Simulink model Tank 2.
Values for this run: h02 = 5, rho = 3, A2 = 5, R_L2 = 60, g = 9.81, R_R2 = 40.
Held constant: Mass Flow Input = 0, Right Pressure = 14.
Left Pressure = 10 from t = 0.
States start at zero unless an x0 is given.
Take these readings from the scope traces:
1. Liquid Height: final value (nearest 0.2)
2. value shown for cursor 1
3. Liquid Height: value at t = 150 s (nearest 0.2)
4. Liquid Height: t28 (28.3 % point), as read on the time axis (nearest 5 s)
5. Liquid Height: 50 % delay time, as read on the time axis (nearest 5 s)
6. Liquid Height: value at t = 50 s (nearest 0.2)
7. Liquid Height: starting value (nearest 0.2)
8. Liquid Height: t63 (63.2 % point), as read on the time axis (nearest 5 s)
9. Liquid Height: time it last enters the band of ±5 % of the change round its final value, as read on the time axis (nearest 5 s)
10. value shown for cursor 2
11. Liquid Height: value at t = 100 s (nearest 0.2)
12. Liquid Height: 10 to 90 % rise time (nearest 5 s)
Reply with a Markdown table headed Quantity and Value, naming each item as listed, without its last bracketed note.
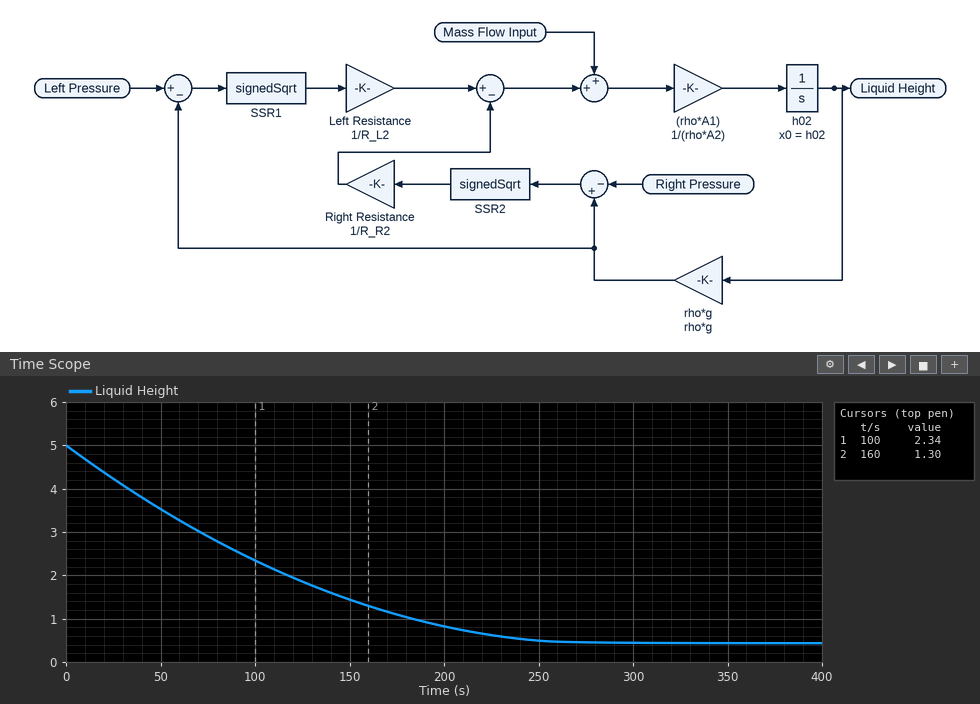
| Quantity | Value |
|---|---|
| Liquid Height: final value | 0.4 |
| value shown for cursor 1 | 2.34 |
| Liquid Height: value at t = 150 s | 1.4 |
| Liquid Height: t28 (28.3 % point), as read on the time axis | 45 s |
| Liquid Height: 50 % delay time, as read on the time axis | 85 s |
| Liquid Height: value at t = 50 s | 3.6 |
| Liquid Height: starting value | 5.0 |
| Liquid Height: t63 (63.2 % point), as read on the time axis | 110 s |
| Liquid Height: time it last enters the band of ±5 % of the change round its final value, as read on the time axis | 220 s |
| value shown for cursor 2 | 1.30 |
| Liquid Height: value at t = 100 s | 2.4 |
| Liquid Height: 10 to 90 % rise time | 180 s |
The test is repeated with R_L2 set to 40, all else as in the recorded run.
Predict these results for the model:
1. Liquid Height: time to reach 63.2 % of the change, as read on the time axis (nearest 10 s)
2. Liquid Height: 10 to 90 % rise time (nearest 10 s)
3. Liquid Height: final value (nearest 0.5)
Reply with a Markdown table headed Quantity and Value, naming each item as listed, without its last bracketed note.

| Quantity | Value |
|---|---|
| Liquid Height: time to reach 63.2 % of the change, as read on the time axis | 90 s |
| Liquid Height: 10 to 90 % rise time | 150 s |
| Liquid Height: final value | 0.5 |
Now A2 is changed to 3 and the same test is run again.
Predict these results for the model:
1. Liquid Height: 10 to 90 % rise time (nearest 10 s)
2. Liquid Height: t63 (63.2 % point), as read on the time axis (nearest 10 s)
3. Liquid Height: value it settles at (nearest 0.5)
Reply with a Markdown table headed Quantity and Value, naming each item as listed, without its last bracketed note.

| Quantity | Value |
|---|---|
| Liquid Height: 10 to 90 % rise time | 110 s |
| Liquid Height: t63 (63.2 % point), as read on the time axis | 70 s |
| Liquid Height: value it settles at | 0.5 |
